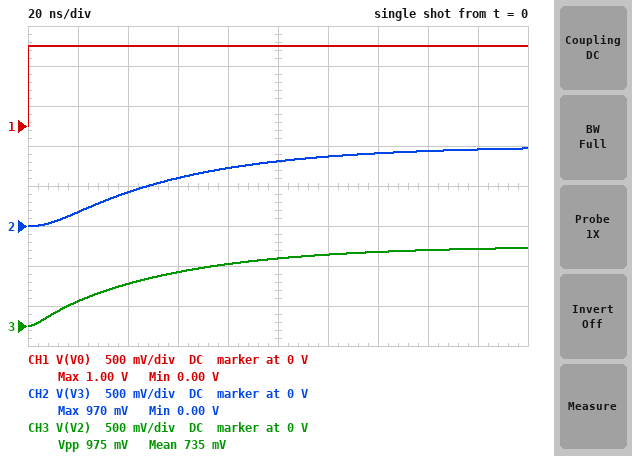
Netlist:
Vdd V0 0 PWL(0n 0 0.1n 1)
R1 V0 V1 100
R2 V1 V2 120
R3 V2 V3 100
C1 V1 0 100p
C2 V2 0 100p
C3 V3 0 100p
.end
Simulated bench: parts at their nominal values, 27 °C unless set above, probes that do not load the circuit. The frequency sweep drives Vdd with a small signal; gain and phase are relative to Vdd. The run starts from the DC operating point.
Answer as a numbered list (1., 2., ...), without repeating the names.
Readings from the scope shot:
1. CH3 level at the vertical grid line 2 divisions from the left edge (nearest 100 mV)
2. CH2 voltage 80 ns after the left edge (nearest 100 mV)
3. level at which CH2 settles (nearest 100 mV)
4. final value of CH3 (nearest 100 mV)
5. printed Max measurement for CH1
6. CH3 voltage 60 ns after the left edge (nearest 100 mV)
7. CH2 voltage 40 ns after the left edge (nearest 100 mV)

1. 500 mV
2. 700 mV
3. 1.0 V
4. 1.0 V
5. 1.00 V
6. 700 mV
7. 400 mV
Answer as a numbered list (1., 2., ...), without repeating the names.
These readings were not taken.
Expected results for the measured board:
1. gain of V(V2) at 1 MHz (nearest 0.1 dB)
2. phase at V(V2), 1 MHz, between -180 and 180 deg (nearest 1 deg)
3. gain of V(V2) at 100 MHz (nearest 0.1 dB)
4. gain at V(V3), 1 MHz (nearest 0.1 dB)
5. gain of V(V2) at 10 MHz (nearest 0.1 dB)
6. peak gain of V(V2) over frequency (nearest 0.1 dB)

1. -0.5 dB
2. -19 deg
3. -34.5 dB
4. -0.5 dB
5. -10.4 dB
6. 0 dB
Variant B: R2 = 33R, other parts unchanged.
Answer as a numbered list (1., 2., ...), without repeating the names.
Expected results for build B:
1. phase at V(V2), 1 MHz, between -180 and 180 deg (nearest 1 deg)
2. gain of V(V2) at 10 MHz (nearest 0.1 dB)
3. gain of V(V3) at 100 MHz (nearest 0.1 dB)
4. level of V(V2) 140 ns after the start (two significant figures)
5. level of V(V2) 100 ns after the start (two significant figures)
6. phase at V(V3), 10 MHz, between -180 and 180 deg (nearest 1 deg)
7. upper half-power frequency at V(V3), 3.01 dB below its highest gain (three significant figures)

1. -13 deg
2. -7.7 dB
3. -42.2 dB
4. 970 mV
5. 930 mV
6. -94 deg
7. 3.97 MHz
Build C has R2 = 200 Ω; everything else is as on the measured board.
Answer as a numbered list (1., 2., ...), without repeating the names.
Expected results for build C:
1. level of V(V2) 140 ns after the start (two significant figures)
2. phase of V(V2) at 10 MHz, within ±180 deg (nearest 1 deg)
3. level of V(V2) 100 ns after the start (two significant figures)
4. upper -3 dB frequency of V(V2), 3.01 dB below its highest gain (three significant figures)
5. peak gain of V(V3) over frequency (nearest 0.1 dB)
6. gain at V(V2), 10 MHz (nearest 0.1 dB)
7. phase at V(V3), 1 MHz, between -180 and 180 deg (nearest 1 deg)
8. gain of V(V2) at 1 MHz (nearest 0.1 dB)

1. 870 mV
2. -83 deg
3. 760 mV
4. 2.33 MHz
5. 0 dB
6. -12.6 dB
7. -27 deg
8. -0.7 dB
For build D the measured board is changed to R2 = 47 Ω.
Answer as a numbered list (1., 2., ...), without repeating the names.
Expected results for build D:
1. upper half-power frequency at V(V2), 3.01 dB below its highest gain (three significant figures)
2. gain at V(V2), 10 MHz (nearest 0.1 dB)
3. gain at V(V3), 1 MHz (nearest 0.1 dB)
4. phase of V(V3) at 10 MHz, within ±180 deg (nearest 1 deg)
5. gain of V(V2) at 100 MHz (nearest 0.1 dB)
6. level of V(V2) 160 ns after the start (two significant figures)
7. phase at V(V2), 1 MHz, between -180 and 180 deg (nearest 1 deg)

1. 3.98 MHz
2. -8.1 dB
3. -0.3 dB
4. -97 deg
5. -27.9 dB
6. 980 mV
7. -14 deg
